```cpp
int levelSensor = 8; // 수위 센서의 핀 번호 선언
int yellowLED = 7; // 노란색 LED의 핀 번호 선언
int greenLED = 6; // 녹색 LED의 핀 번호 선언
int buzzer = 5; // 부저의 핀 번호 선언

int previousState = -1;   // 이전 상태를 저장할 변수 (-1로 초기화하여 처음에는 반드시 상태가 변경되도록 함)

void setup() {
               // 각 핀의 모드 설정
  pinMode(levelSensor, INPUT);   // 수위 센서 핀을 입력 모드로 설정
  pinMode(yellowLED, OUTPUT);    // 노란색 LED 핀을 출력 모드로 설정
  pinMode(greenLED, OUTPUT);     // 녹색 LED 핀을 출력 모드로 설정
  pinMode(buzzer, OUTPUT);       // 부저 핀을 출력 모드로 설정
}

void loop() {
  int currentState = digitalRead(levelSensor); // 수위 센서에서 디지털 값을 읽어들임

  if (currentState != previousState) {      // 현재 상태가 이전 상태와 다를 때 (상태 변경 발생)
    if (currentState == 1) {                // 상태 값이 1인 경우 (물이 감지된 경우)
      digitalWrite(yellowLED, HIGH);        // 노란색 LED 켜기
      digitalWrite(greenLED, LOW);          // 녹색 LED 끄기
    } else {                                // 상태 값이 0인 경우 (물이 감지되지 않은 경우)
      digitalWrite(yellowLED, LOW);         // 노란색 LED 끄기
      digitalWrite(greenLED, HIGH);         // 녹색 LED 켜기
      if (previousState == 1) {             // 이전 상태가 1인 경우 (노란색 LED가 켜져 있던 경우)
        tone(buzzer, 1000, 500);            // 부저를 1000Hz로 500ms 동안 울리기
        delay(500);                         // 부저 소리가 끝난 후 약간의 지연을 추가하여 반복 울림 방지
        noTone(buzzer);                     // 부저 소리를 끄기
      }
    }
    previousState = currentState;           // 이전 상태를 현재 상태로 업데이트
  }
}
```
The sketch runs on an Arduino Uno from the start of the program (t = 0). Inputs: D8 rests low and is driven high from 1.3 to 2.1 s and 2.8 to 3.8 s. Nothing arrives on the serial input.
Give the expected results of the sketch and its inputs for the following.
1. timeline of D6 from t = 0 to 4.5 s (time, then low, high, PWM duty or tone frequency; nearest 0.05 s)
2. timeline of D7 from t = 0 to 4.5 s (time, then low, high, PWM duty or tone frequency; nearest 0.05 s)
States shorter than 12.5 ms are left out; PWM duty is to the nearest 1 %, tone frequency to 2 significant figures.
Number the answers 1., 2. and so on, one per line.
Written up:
1. 0 s high; 1.3 s low; 2.1 s high; 2.8 s low; 3.8 s high
2. 0 s low; 1.3 s high; 2.1 s low; 2.8 s high; 3.8 s low
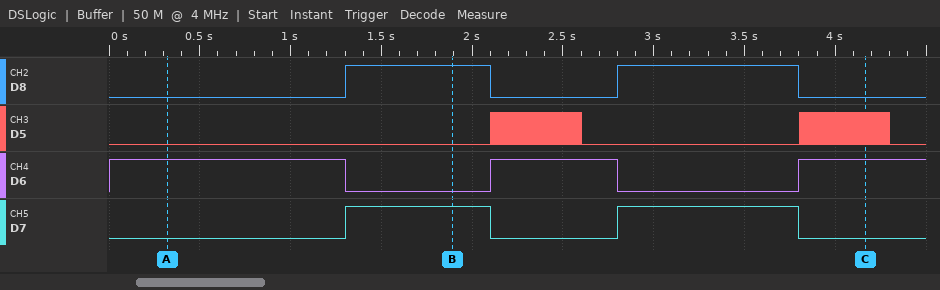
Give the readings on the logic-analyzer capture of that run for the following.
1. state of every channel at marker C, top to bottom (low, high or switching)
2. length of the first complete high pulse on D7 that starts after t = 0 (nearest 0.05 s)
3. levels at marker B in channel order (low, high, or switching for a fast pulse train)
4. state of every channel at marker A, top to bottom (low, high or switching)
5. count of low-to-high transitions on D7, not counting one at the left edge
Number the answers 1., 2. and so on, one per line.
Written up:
1. D8 low, D5 switching, D6 high, D7 low
2. 0.80 s
3. D8 high, D5 low, D6 low, D7 high
4. D8 low, D5 low, D6 high, D7 low
5. 2
